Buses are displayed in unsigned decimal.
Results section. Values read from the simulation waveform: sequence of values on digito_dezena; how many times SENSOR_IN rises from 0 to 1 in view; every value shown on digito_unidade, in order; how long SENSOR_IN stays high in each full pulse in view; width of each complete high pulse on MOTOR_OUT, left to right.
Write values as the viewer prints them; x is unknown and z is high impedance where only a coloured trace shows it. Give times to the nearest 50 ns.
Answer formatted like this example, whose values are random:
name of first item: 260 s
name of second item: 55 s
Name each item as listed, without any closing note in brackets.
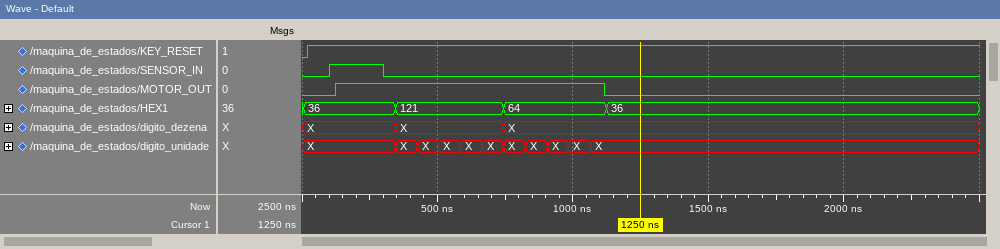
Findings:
sequence of values on digito_dezena: X, X, X
how many times SENSOR_IN rises from 0 to 1 in view: 1
every value shown on digito_unidade, in order: X, X, X, X, X, X, X, X, X, X, X
how long SENSOR_IN stays high in each full pulse in view: 200 ns
width of each complete high pulse on MOTOR_OUT, left to right: 1000 ns
